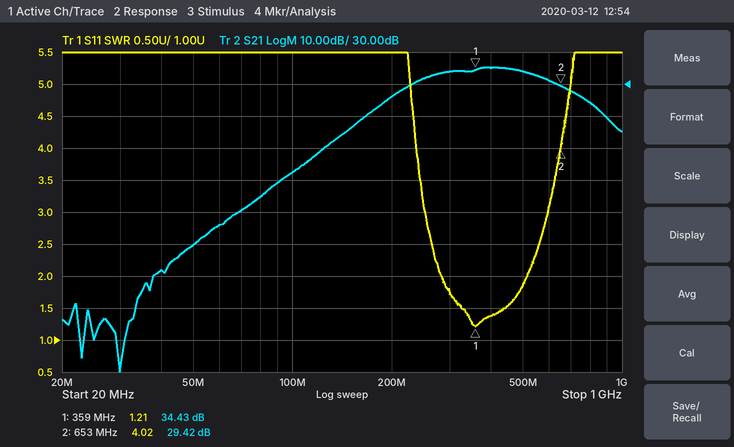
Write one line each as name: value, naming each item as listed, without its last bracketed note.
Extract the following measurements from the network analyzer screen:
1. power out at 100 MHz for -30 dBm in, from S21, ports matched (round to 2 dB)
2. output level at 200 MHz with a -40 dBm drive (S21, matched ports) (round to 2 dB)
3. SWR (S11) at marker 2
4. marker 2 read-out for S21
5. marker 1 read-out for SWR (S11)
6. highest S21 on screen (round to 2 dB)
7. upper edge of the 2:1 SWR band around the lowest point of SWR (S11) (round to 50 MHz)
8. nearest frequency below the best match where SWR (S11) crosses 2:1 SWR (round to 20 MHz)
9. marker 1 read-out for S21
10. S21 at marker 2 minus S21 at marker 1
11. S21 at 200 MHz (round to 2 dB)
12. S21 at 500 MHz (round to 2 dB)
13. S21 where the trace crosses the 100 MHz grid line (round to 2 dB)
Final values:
power out at 100 MHz for -30 dBm in, from S21, ports matched: -28 dBm
output level at 200 MHz with a -40 dBm drive (S21, matched ports): -14 dBm
SWR (S11) at marker 2: 4.02
marker 2 read-out for S21: 29.42 dB
marker 1 read-out for SWR: 1.21
highest S21 on screen: 36 dB
upper edge of the 2:1 SWR band around the lowest point of SWR (S11): 500 MHz
nearest frequency below the best match where SWR (S11) crosses 2:1 SWR: 280 MHz
marker 1 read-out for S21: 34.43 dB
S21 at marker 2 minus S21 at marker 1: -5.01 dB
S21 at 200 MHz: 26 dB
S21 at 500 MHz: 34 dB
S21 where the trace crosses the 100 MHz grid line: 2 dB
